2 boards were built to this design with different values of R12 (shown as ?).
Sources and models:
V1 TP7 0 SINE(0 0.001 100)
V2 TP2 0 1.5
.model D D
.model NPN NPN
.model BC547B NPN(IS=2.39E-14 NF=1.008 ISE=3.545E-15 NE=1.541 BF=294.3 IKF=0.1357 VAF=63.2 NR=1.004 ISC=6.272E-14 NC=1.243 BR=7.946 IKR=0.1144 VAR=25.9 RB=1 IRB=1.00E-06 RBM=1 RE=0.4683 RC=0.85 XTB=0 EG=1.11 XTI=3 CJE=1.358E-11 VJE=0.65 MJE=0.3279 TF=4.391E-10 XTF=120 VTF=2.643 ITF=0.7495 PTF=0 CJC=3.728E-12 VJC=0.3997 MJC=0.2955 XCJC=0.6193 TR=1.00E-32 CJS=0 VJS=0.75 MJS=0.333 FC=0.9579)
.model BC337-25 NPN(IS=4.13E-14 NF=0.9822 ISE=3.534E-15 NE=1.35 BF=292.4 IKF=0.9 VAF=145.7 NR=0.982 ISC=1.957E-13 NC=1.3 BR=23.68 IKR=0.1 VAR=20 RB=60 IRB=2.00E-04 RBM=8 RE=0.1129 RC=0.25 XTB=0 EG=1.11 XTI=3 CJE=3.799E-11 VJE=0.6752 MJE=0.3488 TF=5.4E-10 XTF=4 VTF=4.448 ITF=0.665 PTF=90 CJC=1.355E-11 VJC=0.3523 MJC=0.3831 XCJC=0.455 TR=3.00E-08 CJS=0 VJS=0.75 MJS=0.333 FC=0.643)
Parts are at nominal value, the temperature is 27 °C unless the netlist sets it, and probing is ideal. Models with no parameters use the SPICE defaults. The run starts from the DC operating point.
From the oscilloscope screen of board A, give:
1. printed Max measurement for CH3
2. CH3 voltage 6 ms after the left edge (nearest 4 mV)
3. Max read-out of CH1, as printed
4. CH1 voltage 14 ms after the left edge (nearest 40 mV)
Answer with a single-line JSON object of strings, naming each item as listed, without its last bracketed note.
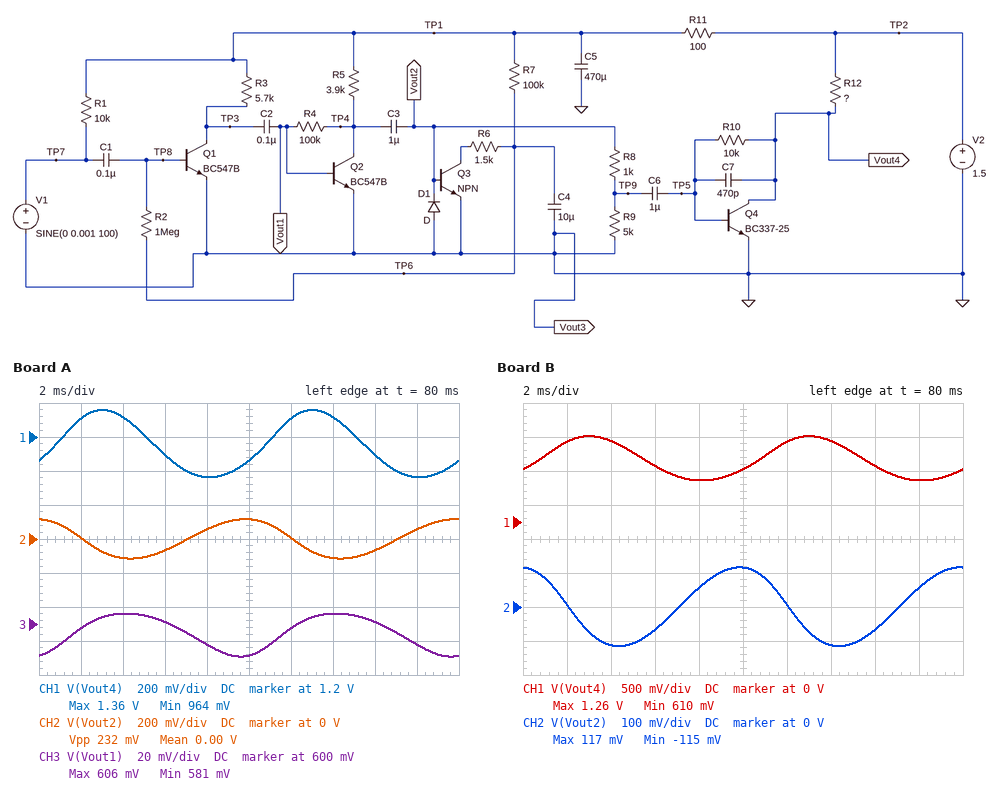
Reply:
{"printed Max measurement for CH3": "606 mV", "CH3 voltage 6 ms after the left edge": "600 mV", "Max read-out of CH1, as printed": "1.36 V", "CH1 voltage 14 ms after the left edge": "1.32 V"}
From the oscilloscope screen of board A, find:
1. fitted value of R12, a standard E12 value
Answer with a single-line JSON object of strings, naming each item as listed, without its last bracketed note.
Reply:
{"fitted value of R12, a standard E12 value": "27 Ω"}
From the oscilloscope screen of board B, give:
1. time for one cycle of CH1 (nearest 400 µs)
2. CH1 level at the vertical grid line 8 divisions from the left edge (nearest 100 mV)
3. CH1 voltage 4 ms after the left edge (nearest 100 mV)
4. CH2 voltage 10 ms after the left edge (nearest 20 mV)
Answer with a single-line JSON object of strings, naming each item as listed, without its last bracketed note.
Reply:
{"time for one cycle of CH1": "10.0 ms", "CH1 level at the vertical grid line 8 divisions from the left edge": "800 mV", "CH1 voltage 4 ms after the left edge": "1.2 V", "CH2 voltage 10 ms after the left edge": "120 mV"}
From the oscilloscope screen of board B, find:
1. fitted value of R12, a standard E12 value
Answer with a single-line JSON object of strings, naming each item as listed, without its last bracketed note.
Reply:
{"fitted value of R12, a standard E12 value": "82 Ω"}
